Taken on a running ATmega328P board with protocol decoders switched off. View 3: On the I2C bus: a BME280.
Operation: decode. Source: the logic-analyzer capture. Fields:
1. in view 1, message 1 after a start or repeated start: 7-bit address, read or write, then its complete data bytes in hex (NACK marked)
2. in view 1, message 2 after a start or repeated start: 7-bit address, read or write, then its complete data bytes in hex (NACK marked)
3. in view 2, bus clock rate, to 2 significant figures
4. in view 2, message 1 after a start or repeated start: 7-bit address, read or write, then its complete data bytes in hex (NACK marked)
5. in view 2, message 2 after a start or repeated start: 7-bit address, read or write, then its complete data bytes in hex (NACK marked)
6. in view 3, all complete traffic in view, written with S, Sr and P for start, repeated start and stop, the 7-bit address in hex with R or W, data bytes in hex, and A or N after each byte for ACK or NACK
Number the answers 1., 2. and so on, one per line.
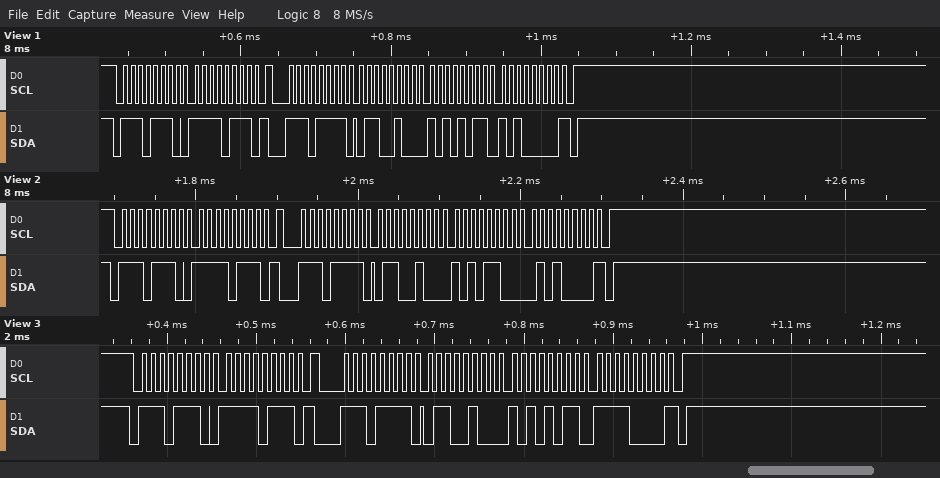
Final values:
1. 0x77 write: F7
2. 0x77 read: 64 AB A0 NACK
3. 100 kHz
4. 0x77 write: F7
5. 0x77 read: 64 AC 50 NACK
6. S 77W A F7 A Sr 77R A 64 A AB A F0 N P
